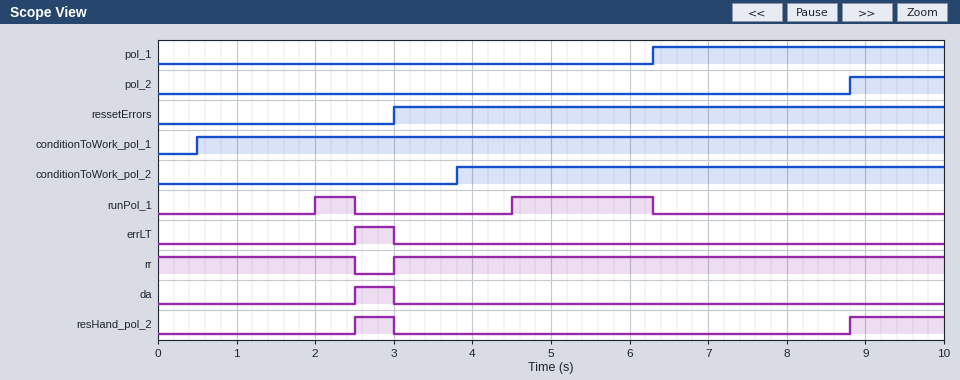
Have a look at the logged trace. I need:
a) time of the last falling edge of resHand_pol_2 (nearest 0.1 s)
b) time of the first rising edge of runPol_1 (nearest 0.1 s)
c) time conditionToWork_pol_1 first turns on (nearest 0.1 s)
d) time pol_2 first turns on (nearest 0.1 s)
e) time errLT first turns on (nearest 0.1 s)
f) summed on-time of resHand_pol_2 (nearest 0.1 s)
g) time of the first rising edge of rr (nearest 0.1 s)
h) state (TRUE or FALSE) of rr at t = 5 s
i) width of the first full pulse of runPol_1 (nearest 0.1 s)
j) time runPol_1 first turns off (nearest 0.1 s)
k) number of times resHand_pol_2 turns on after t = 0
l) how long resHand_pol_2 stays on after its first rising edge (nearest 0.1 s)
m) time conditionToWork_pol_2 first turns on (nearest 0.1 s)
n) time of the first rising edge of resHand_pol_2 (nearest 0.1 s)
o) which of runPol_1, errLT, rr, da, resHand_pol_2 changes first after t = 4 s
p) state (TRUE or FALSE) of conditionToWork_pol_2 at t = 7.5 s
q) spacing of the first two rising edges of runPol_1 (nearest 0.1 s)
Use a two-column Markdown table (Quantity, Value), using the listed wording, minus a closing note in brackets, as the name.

| Quantity | Value |
|---|---|
| time of the last falling edge of resHand_pol_2 | 3.0 s |
| time of the first rising edge of runPol_1 | 2.0 s |
| time conditionToWork_pol_1 first turns on | 0.5 s |
| time pol_2 first turns on | 8.8 s |
| time errLT first turns on | 2.5 s |
| summed on-time of resHand_pol_2 | 1.7 s |
| time of the first rising edge of rr | 3.0 s |
| state (TRUE or FALSE) of rr at t = 5 s | TRUE |
| width of the first full pulse of runPol_1 | 0.5 s |
| time runPol_1 first turns off | 2.5 s |
| number of times resHand_pol_2 turns on after t = 0 | 2 |
| how long resHand_pol_2 stays on after its first rising edge | 0.5 s |
| time conditionToWork_pol_2 first turns on | 3.8 s |
| time of the first rising edge of resHand_pol_2 | 2.5 s |
| which of runPol_1, errLT, rr, da, resHand_pol_2 changes first after t = 4 s | runPol_1 |
| state (TRUE or FALSE) of conditionToWork_pol_2 at t = 7.5 s | TRUE |
| spacing of the first two rising edges of runPol_1 | 2.5 s |
